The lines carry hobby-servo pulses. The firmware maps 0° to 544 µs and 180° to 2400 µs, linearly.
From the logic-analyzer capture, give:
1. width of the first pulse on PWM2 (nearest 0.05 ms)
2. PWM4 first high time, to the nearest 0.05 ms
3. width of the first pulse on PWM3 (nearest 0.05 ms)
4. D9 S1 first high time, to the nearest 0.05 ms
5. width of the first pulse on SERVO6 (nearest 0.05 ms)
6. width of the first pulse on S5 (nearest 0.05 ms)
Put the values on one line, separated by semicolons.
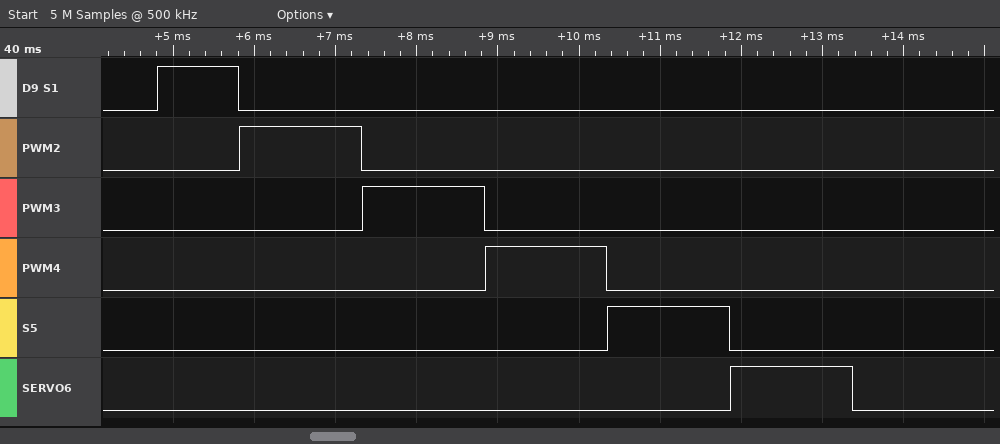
1.50 ms; 1.50 ms; 1.50 ms; 1.00 ms; 1.50 ms; 1.50 ms
